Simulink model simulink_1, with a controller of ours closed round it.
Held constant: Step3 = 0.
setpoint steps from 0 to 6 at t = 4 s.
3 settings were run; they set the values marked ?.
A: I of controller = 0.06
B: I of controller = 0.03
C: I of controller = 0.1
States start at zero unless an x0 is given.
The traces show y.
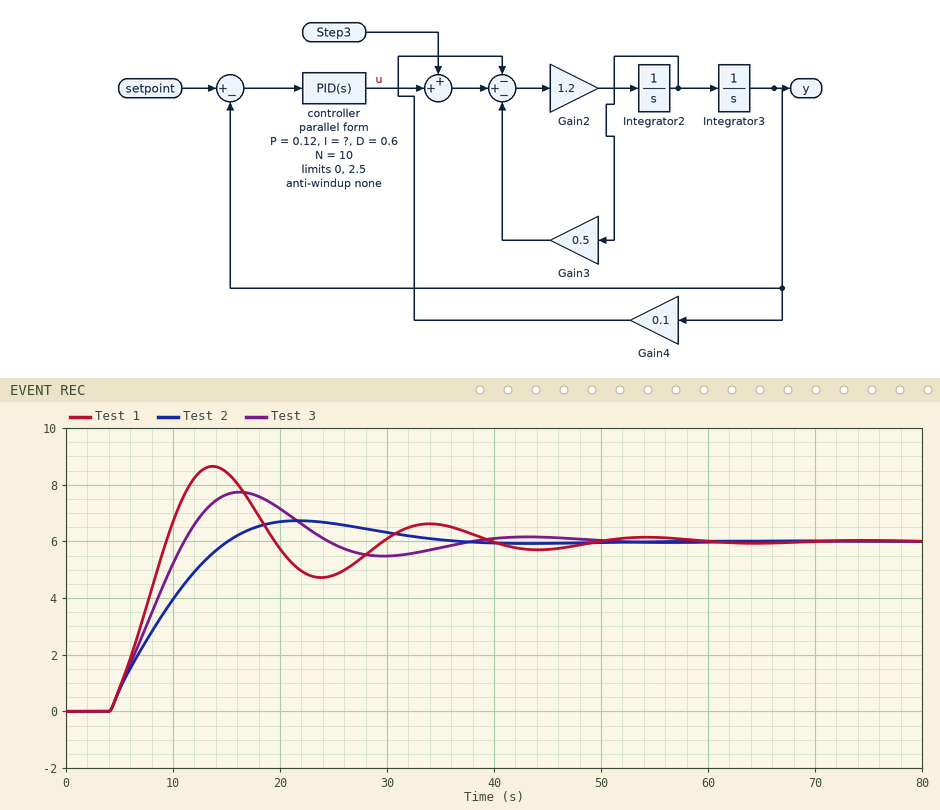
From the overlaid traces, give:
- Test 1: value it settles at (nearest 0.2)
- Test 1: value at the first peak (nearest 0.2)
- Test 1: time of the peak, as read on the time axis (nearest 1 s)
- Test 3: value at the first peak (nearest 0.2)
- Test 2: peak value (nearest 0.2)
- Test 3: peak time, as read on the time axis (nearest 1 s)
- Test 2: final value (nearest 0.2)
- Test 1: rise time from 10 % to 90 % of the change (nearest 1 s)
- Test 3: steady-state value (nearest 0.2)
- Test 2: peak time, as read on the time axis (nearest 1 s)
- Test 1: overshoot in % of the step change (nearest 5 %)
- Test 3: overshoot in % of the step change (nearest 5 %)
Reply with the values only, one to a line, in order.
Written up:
6.0
8.6
14 s
7.8
6.8
16 s
6.0
4 s
6.0
22 s
45 %
30 %
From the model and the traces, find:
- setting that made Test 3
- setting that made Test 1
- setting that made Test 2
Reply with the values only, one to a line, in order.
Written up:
A
C
B
